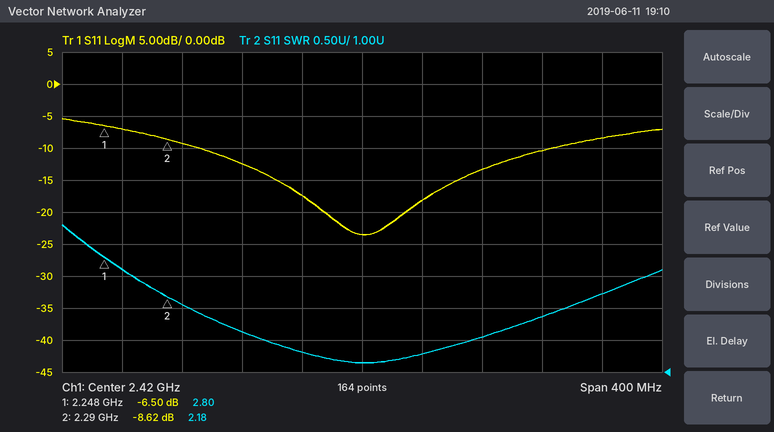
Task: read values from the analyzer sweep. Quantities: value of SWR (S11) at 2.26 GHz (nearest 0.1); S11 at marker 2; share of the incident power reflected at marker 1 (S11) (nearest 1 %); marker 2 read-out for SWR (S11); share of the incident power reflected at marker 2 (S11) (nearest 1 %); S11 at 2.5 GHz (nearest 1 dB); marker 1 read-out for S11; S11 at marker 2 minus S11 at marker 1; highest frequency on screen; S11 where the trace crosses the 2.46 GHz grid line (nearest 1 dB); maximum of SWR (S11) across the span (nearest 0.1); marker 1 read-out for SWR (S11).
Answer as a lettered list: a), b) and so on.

a) 2.6
b) -8.62 dB
c) 22 %
d) 2.18
e) 14 %
f) -13 dB
g) -6.50 dB
h) -2.12 dB
i) 2.62 GHz
j) -18 dB
k) 3.3
l) 2.80
